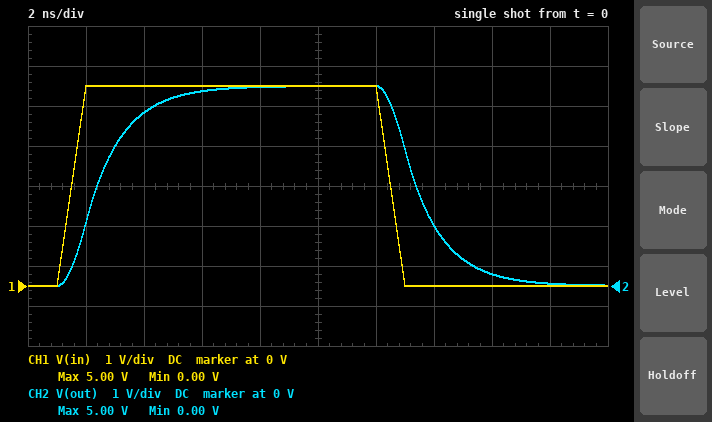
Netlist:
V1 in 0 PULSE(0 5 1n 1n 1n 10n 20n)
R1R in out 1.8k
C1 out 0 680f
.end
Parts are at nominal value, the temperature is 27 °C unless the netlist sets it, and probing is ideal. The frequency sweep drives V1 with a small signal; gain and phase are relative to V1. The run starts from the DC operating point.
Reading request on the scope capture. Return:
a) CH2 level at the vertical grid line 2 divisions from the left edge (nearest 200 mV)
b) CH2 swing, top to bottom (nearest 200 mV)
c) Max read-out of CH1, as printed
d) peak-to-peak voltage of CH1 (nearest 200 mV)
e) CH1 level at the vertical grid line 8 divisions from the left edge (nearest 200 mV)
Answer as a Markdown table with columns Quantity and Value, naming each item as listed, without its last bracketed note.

| Quantity | Value |
|---|---|
| CH2 level at the vertical grid line 2 divisions from the left edge | 4.4 V |
| CH2 swing, top to bottom | 5.0 V |
| Max read-out of CH1, as printed | 5.00 V |
| peak-to-peak voltage of CH1 | 5.0 V |
| CH1 level at the vertical grid line 8 divisions from the left edge | 0 V |
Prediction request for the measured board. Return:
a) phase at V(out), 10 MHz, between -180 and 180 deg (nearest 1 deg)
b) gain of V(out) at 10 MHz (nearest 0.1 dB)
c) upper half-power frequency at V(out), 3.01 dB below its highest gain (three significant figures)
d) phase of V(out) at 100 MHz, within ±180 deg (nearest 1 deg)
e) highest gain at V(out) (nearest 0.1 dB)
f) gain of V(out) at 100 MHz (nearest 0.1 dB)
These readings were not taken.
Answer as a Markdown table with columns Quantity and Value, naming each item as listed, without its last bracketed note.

| Quantity | Value |
|---|---|
| phase at V(out), 10 MHz, between -180 and 180 deg | -4 deg |
| gain of V(out) at 10 MHz | 0 dB |
| upper half-power frequency at V(out), 3.01 dB below its highest gain | 130 MHz |
| phase of V(out) at 100 MHz, within ±180 deg | -38 deg |
| highest gain at V(out) | 0 dB |
| gain of V(out) at 100 MHz | -2.0 dB |
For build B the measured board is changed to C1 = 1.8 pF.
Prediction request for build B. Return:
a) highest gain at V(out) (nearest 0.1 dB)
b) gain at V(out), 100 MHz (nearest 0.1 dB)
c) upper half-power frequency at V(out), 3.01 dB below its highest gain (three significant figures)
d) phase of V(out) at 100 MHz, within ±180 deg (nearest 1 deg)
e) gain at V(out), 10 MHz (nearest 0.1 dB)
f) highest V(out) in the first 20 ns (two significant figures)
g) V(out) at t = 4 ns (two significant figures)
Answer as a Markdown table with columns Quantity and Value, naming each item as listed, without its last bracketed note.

| Quantity | Value |
|---|---|
| highest gain at V(out) | 0 dB |
| gain at V(out), 100 MHz | -7.1 dB |
| upper half-power frequency at V(out), 3.01 dB below its highest gain | 49.1 MHz |
| phase of V(out) at 100 MHz, within ±180 deg | -64 deg |
| gain at V(out), 10 MHz | -0.2 dB |
| highest V(out) in the first 20 ns | 4.8 V |
| V(out) at t = 4 ns | 2.7 V |
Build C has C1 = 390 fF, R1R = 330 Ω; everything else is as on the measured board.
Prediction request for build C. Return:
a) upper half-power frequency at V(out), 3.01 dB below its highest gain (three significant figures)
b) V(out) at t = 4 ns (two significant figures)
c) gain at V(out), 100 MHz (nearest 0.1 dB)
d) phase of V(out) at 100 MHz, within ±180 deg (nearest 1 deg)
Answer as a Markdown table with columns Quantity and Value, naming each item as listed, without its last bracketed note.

| Quantity | Value |
|---|---|
| upper half-power frequency at V(out), 3.01 dB below its highest gain | 1.24 GHz |
| V(out) at t = 4 ns | 5.0 V |
| gain at V(out), 100 MHz | 0 dB |
| phase of V(out) at 100 MHz, within ±180 deg | -5 deg |
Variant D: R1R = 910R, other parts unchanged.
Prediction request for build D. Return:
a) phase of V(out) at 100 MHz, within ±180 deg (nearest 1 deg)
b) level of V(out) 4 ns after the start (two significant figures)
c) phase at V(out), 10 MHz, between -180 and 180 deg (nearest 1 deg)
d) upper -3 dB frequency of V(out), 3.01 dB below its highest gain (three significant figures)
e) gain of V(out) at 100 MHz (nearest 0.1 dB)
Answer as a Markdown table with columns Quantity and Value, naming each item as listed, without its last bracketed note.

| Quantity | Value |
|---|---|
| phase of V(out) at 100 MHz, within ±180 deg | -21 deg |
| level of V(out) 4 ns after the start | 4.9 V |
| phase at V(out), 10 MHz, between -180 and 180 deg | -2 deg |
| upper -3 dB frequency of V(out), 3.01 dB below its highest gain | 257 MHz |
| gain of V(out) at 100 MHz | -0.6 dB |
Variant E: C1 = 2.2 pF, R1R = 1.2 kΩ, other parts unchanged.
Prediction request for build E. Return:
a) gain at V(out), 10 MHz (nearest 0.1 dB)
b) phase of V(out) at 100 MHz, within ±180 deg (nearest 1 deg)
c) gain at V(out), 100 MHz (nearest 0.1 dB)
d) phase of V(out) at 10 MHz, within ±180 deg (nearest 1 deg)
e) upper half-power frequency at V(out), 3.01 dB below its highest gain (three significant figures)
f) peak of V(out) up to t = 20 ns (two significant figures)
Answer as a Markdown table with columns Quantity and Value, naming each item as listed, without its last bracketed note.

| Quantity | Value |
|---|---|
| gain at V(out), 10 MHz | -0.1 dB |
| phase of V(out) at 100 MHz, within ±180 deg | -59 deg |
| gain at V(out), 100 MHz | -5.7 dB |
| phase of V(out) at 10 MHz, within ±180 deg | -9 deg |
| upper half-power frequency at V(out), 3.01 dB below its highest gain | 60.3 MHz |
| peak of V(out) up to t = 20 ns | 4.9 V |
